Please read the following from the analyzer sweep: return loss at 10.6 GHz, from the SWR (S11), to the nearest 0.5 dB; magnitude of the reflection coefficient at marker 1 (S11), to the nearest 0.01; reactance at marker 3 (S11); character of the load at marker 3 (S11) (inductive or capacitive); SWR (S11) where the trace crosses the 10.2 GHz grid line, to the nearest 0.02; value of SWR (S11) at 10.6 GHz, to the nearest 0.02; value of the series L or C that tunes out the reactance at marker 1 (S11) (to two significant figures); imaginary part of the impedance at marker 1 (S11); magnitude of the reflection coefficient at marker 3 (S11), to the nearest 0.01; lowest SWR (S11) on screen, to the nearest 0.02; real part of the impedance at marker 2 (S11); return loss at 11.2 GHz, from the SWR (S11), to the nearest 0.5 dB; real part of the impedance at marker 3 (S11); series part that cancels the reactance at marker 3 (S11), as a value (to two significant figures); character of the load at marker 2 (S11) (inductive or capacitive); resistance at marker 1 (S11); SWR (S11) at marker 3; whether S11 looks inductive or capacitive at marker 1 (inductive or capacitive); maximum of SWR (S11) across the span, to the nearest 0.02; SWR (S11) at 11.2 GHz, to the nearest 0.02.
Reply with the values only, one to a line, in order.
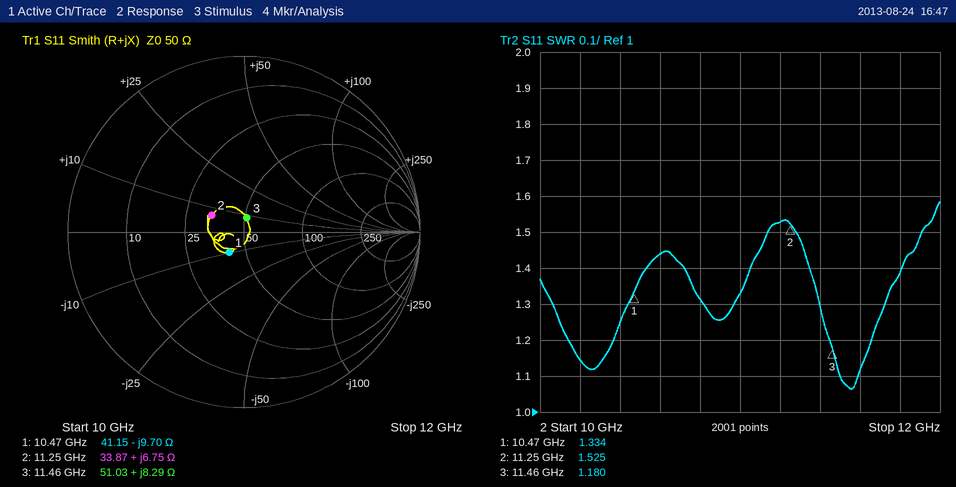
15.0 dB
0.14
+8.29 Ω
inductive
1.14
1.44
150 pH
-9.70 Ω
0.08
1.06
33.87 Ω
13.5 dB
51.03 Ω
1.7 pF
inductive
41.15 Ω
1.180
capacitive
1.58
1.52
